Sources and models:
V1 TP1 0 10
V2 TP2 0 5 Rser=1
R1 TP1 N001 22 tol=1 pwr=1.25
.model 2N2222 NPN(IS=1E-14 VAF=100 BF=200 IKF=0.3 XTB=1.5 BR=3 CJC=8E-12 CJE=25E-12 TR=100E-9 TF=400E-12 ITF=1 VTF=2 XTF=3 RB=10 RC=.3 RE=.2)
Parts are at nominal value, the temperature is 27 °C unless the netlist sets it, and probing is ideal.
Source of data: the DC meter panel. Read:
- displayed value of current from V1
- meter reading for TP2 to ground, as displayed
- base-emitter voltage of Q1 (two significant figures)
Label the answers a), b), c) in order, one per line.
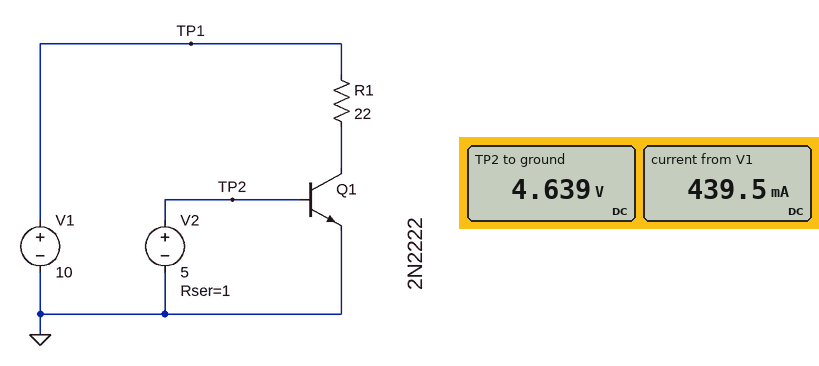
a) 439.5 mA
b) 4.639 V
c) 4.6 V
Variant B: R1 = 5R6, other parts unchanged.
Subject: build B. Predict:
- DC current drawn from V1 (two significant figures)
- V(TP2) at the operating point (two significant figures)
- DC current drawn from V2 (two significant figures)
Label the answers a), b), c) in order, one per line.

a) 1.6 A
b) 4.7 V
c) 340 mA
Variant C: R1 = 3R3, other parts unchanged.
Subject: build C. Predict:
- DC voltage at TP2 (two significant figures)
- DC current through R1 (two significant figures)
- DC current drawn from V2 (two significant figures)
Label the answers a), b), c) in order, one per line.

a) 4.7 V
b) 2.6 A
c) 320 mA
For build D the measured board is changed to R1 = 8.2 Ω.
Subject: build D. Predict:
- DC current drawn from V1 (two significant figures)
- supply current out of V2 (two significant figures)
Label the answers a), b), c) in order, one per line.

a) 1.1 A
b) 350 mA
